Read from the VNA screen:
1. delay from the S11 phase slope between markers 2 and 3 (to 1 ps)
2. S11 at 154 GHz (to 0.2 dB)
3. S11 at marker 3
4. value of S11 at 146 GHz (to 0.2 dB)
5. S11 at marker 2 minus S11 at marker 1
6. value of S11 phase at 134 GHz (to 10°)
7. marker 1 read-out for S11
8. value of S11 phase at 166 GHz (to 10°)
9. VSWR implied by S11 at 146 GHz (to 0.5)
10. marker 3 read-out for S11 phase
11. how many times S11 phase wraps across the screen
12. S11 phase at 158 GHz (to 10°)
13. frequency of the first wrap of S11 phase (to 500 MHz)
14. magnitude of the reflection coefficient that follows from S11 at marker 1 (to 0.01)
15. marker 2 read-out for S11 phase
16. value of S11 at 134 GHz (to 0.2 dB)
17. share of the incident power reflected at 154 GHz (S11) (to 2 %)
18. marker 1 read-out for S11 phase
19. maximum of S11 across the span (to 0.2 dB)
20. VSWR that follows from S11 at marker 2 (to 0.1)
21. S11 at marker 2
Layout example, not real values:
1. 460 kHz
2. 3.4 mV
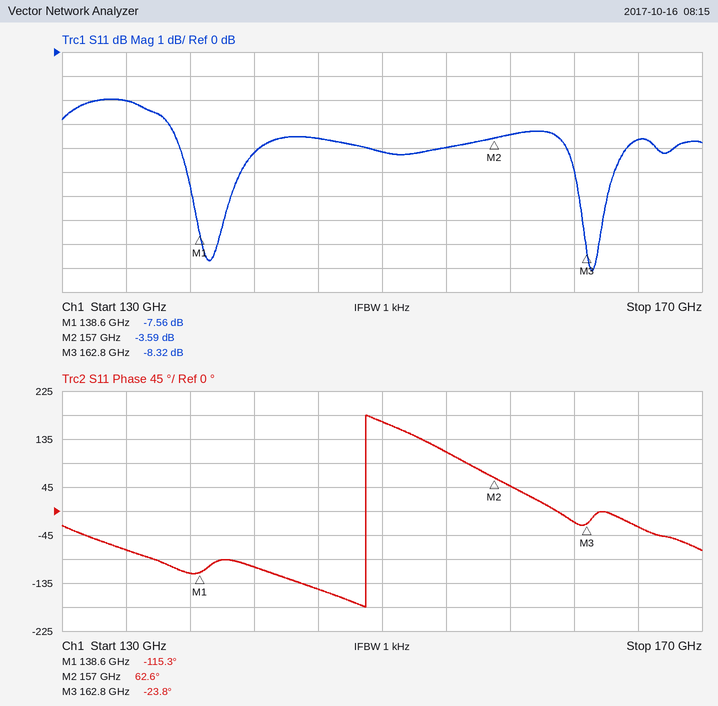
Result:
1. 41 ps
2. -4.0 dB
3. -8.32 dB
4. -3.6 dB
5. 3.97 dB
6. -70°
7. -7.56 dB
8. -30°
9. 5.0
10. -23.8°
11. 1
12. 50°
13. 149.0 GHz
14. 0.42
15. 62.6°
16. -2.0 dB
17. 40 %
18. -115.3°
19. -2.0 dB
20. 4.9
21. -3.59 dB
